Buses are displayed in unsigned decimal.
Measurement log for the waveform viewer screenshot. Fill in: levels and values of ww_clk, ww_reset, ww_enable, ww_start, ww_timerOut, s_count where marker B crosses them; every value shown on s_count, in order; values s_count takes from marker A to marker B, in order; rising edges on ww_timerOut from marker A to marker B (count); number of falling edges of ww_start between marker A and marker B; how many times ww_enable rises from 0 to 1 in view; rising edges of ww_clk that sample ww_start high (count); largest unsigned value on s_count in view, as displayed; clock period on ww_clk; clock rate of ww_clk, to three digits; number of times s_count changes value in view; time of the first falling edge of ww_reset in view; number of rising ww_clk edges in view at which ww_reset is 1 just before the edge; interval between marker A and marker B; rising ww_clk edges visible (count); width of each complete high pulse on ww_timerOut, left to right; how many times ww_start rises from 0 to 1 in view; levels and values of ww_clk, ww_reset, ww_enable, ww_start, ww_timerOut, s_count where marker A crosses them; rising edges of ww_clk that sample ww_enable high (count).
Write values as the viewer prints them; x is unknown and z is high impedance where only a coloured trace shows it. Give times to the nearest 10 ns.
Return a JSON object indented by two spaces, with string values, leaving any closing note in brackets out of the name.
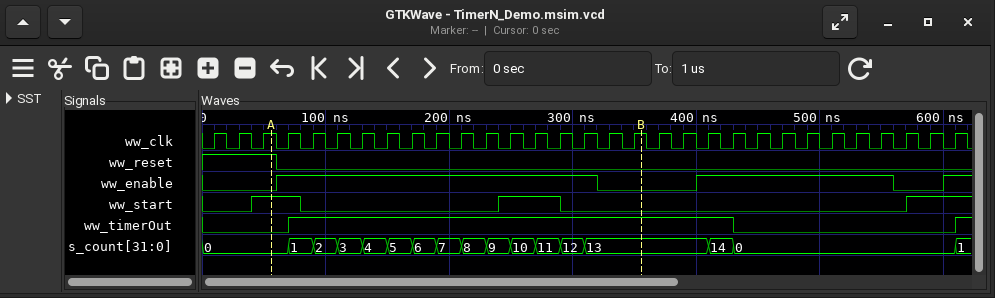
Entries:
{
  "levels and values of ww_clk, ww_reset, ww_enable, ww_start, ww_timerOut, s_count where marker B crosses them": "ww_clk=1, ww_reset=0, ww_enable=0, ww_start=0, ww_timerOut=1, s_count=13",
  "every value shown on s_count, in order": "0, 1, 2, 3, 4, 5, 6, 7, 8, 9, 10, 11, 12, 13, 14, 0, 1",
  "values s_count takes from marker A to marker B, in order": "0, 1, 2, 3, 4, 5, 6, 7, 8, 9, 10, 11, 12, 13",
  "rising edges on ww_timerOut from marker A to marker B": "1",
  "number of falling edges of ww_start between marker A and marker B": "2",
  "how many times ww_enable rises from 0 to 1 in view": "3",
  "rising edges of ww_clk that sample ww_start high": "7",
  "largest unsigned value on s_count in view, as displayed": "14",
  "clock period on ww_clk": "20 ns",
  "clock rate of ww_clk, to three digits": "50.0 MHz",
  "number of times s_count changes value in view": "16",
  "time of the first falling edge of ww_reset in view": "60 ns",
  "number of rising ww_clk edges in view at which ww_reset is 1 just before the edge": "3",
  "interval between marker A and marker B": "300 ns",
  "rising ww_clk edges visible": "31",
  "width of each complete high pulse on ww_timerOut, left to right": "360 ns",
  "how many times ww_start rises from 0 to 1 in view": "3",
  "levels and values of ww_clk, ww_reset, ww_enable, ww_start, ww_timerOut, s_count where marker A crosses them": "ww_clk=1, ww_reset=1, ww_enable=0, ww_start=1, ww_timerOut=0, s_count=0",
  "rising edges of ww_clk that sample ww_enable high": "22"
}
